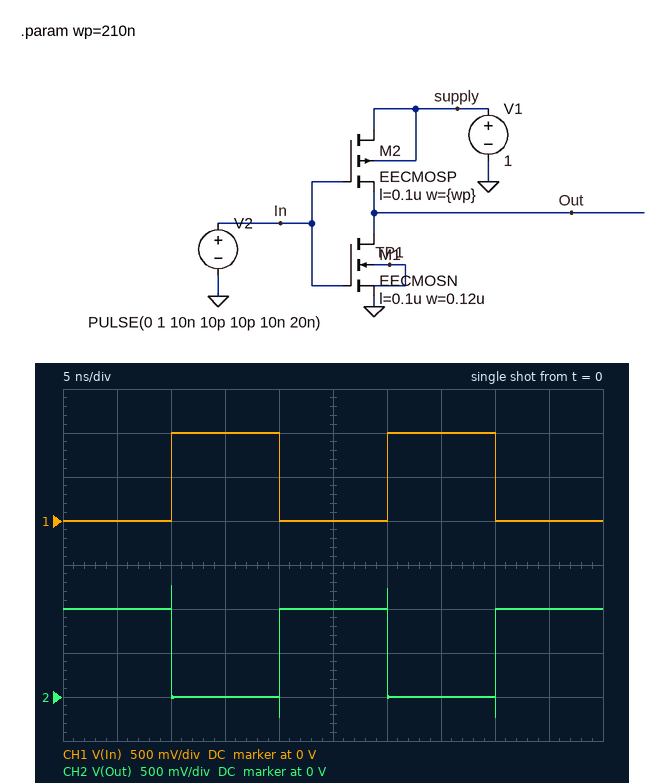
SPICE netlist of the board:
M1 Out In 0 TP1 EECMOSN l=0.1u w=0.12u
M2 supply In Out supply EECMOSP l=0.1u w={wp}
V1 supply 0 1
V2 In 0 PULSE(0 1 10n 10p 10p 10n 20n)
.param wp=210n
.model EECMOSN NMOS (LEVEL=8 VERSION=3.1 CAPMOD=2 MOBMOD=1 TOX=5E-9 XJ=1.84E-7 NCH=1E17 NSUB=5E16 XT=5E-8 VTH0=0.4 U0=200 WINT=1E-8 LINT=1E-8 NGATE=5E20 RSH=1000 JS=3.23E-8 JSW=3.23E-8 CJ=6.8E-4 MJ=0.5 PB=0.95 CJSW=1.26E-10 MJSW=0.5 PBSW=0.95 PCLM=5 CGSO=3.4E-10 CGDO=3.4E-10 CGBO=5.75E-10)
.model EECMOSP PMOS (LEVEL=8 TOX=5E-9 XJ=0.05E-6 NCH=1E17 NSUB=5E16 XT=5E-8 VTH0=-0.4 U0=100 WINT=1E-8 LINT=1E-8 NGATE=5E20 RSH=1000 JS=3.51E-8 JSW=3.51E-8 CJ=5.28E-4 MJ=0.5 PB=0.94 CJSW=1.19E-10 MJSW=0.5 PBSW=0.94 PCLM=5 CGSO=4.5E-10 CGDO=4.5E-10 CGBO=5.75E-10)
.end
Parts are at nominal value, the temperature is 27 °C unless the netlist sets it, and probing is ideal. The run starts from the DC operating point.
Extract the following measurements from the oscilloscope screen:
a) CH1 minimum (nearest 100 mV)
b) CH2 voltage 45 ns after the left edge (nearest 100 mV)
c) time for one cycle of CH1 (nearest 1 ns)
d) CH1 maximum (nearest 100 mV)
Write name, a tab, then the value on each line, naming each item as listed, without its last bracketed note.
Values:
CH1 minimum	0 V
CH2 voltage 45 ns after the left edge	1.0 V
time for one cycle of CH1	20 ns
CH1 maximum	1.0 V
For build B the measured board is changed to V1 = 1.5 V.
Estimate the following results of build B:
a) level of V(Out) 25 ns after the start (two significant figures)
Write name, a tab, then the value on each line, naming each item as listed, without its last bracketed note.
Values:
level of V(Out) 25 ns after the start	1.5 V
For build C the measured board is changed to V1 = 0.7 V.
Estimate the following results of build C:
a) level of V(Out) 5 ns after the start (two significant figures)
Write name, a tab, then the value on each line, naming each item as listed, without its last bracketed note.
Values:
level of V(Out) 5 ns after the start	700 mV
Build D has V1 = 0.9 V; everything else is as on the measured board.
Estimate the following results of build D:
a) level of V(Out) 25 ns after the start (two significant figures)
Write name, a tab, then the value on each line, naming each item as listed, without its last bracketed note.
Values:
level of V(Out) 25 ns after the start	900 mV
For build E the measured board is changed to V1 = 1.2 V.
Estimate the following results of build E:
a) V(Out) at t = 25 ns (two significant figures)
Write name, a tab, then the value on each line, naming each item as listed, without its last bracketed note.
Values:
V(Out) at t = 25 ns	1.2 V
